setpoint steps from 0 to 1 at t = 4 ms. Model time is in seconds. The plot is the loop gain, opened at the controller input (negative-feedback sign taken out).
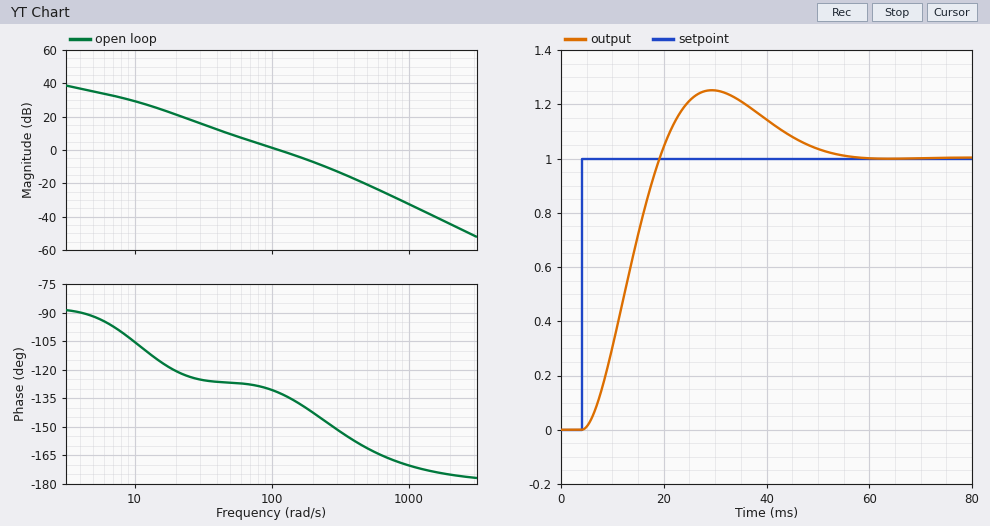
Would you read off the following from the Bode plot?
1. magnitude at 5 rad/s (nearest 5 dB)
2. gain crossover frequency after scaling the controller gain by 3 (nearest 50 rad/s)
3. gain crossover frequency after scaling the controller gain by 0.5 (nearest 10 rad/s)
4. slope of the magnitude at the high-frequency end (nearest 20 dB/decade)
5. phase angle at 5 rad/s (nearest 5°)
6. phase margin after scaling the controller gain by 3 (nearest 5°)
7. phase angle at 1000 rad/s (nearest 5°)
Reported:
35 dB
250 rad/s
70 rad/s
-40 dB/decade
-90°
35°
-170°
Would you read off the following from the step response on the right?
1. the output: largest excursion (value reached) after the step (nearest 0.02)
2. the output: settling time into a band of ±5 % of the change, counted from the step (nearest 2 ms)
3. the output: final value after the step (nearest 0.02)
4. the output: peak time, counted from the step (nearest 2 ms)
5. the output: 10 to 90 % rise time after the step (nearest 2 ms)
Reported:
1.26
44 ms
1.00
26 ms
10 ms
